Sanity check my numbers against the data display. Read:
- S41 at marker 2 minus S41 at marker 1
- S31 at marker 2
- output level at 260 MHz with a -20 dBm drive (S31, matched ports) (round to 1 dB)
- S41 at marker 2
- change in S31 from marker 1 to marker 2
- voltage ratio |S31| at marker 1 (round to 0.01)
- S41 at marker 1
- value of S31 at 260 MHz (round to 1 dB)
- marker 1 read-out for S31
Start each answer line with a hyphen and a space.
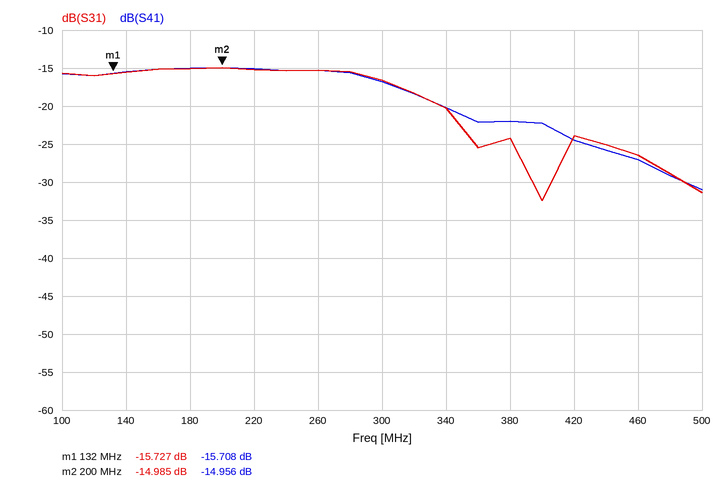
- 0.752 dB
- -14.985 dB
- -35 dBm
- -14.956 dB
- 0.742 dB
- 0.16
- -15.708 dB
- -15 dB
- -15.727 dB
